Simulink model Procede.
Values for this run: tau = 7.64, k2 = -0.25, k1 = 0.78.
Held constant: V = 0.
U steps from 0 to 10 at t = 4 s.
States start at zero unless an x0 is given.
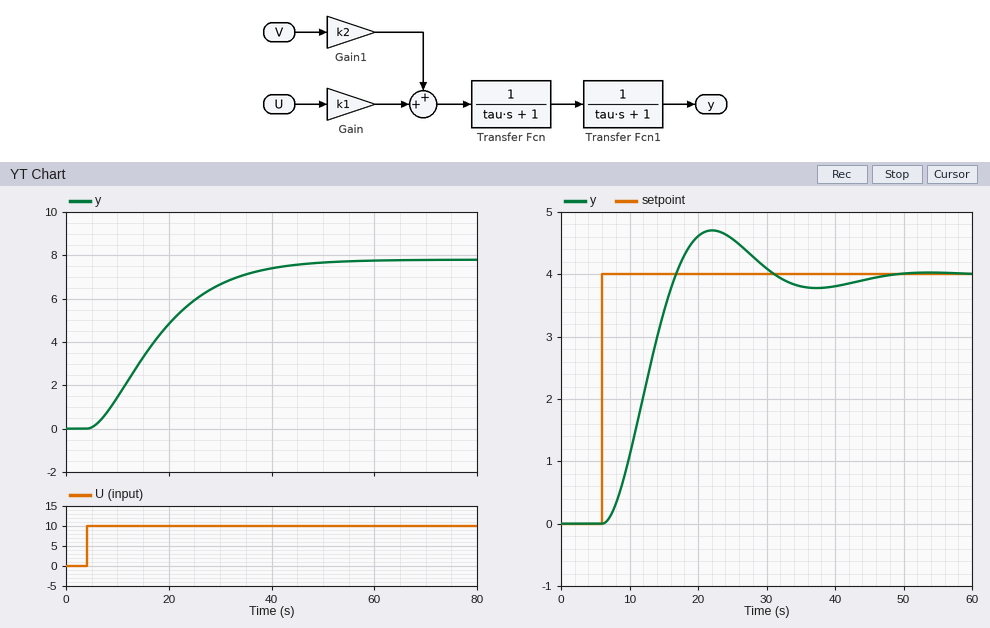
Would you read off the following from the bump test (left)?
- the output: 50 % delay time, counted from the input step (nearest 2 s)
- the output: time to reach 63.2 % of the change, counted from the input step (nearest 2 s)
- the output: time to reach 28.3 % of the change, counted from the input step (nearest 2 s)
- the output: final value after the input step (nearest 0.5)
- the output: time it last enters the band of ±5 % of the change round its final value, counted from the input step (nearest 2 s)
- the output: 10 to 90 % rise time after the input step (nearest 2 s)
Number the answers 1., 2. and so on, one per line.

1. 12 s
2. 16 s
3. 8 s
4. 8.0
5. 36 s
6. 26 s
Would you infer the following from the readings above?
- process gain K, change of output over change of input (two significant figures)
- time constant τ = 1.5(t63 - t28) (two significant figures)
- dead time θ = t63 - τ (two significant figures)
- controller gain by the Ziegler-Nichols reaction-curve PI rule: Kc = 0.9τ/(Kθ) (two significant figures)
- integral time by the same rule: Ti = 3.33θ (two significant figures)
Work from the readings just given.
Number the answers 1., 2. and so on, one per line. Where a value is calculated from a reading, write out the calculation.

1. (8 - 0) / 10 = 0.80
2. 1.5 × (16 - 8) = 12 s
3. 16 - 12 = 4.0 s
4. 0.9 × 12 / (0.8 × 4) = 3.4
5. 3.33 × 4 = 13 s
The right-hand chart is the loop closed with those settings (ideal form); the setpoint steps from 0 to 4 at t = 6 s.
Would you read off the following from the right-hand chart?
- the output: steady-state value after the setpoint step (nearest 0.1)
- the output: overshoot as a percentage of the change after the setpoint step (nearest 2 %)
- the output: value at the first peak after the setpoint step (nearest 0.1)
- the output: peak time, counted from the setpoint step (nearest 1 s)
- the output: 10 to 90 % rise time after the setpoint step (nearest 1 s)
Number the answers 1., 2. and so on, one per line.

1. 4.0
2. 18 %
3. 4.7
4. 16 s
5. 7 s
